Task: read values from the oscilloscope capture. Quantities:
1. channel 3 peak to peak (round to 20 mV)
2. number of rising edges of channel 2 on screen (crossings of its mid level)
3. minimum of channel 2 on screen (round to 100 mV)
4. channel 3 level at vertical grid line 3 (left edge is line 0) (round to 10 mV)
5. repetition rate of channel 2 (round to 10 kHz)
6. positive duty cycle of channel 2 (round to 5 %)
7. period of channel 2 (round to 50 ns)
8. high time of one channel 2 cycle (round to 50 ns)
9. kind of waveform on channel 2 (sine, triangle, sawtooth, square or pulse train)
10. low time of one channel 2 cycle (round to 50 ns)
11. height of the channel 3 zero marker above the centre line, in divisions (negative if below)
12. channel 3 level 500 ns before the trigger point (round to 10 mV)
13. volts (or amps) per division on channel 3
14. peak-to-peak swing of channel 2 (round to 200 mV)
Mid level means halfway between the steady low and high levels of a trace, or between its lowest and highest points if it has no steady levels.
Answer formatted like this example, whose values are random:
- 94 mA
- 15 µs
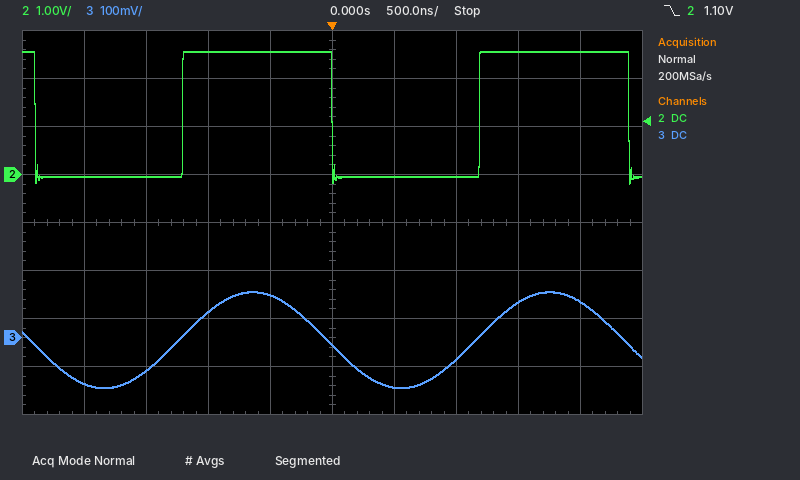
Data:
- 200 mV
- 2
- -200 mV
- 50 mV
- 420 kHz
- 50 %
- 2.40 µs
- 1.20 µs
- square
- 1.20 µs
- -2.4 div
- 90 mV
- 100 mV
- 2.8 V
